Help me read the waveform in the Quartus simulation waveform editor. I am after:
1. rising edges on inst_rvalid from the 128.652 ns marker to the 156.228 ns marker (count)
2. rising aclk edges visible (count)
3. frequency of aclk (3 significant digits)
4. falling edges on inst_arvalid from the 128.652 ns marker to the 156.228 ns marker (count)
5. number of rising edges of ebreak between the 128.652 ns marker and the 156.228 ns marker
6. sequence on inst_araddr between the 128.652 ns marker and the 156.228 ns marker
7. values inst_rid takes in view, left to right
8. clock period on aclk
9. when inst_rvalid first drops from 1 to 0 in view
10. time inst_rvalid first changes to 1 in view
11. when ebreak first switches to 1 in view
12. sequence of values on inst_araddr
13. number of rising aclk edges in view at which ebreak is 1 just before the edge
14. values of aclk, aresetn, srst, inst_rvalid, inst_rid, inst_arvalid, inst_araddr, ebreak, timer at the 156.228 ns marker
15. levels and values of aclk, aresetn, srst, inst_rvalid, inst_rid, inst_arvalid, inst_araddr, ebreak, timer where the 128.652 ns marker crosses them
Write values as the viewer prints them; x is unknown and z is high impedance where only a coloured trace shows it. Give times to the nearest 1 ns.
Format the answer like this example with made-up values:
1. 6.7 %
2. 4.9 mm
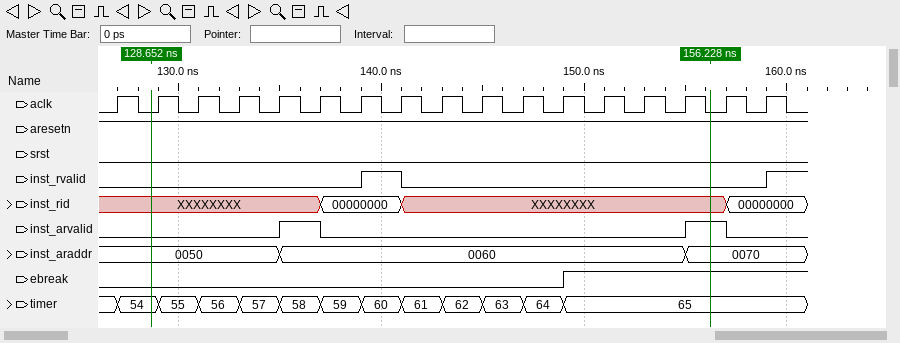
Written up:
1. 1
2. 17
3. 500 MHz
4. 1
5. 1
6. 0050, 0060, 0070
7. XXXXXXXX, 00000000, XXXXXXXX, 00000000
8. 2 ns
9. 141 ns
10. 139 ns
11. 149 ns
12. 0050, 0060, 0070
13. 5
14. aclk=0, aresetn=1, srst=0, inst_rvalid=0, inst_rid=XXXXXXXX, inst_arvalid=1, inst_araddr=0070, ebreak=1, timer=65
15. aclk=0, aresetn=1, srst=0, inst_rvalid=0, inst_rid=XXXXXXXX, inst_arvalid=0, inst_araddr=0050, ebreak=0, timer=54
